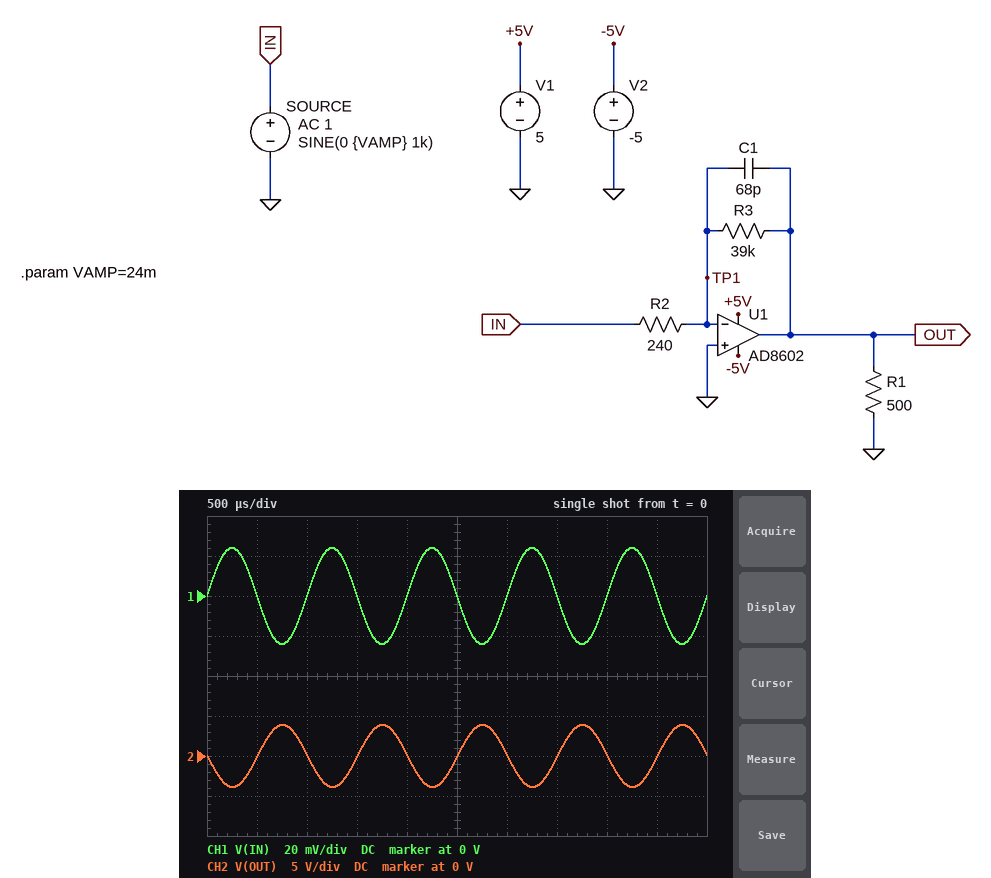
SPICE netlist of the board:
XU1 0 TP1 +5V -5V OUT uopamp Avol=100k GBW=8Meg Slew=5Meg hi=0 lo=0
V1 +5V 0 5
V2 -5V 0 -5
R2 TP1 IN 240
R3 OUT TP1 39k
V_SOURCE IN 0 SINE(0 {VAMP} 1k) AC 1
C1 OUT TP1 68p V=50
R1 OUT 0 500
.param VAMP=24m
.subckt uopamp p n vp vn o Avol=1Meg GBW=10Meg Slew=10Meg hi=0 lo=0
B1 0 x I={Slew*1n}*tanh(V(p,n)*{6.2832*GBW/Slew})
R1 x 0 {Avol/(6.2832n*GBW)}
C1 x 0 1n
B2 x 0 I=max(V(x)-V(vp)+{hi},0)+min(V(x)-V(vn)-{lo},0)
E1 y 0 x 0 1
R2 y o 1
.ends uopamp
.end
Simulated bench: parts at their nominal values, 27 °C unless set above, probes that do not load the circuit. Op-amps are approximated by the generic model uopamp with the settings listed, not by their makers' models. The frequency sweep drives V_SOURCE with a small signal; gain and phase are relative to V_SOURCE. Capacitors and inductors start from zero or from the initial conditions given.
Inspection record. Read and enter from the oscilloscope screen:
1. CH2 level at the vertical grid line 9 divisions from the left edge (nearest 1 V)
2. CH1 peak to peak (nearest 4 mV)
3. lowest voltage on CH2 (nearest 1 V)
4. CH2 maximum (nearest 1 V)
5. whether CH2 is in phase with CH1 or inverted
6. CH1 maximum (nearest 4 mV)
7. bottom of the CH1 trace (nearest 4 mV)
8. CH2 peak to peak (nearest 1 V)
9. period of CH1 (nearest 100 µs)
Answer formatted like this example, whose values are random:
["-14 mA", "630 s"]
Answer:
["0 V", "48 mV", "-4 V", "4 V", "inverted", "24 mV", "-24 mV", "8 V", "1.0 ms"]
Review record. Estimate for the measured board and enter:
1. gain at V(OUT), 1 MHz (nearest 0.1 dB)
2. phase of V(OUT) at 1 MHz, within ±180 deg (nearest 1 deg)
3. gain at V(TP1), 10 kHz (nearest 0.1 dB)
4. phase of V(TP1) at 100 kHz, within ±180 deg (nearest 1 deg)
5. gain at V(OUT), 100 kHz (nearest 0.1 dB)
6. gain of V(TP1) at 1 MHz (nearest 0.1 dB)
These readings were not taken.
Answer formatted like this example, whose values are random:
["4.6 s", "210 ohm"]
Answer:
["12.8 dB", "88 deg", "-14.4 dB", "15 deg", "32.5 dB", "-5.2 dB"]
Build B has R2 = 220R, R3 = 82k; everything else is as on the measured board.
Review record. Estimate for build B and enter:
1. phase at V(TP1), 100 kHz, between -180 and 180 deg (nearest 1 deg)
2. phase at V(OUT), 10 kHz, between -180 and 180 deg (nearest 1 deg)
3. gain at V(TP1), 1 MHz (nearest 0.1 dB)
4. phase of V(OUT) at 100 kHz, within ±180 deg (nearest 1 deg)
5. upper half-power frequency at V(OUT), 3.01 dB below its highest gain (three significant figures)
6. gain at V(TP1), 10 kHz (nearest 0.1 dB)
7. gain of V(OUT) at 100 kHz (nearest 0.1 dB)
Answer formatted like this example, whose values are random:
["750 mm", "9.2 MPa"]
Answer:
["7 deg", "141 deg", "-4.9 dB", "97 deg", "12.3 kHz", "-8.9 dB", "33.1 dB"]
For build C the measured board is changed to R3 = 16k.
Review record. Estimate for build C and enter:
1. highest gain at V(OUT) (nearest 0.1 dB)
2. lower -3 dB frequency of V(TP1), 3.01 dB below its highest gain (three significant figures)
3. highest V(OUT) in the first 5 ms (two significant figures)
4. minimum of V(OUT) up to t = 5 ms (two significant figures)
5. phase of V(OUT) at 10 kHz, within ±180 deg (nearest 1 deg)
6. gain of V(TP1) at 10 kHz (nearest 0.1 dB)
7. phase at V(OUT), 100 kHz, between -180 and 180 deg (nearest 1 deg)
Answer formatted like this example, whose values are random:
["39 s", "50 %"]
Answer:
["36.5 dB", "65.1 kHz", "1.6 V", "-1.6 V", "171 deg", "-21.7 dB", "123 deg"]
